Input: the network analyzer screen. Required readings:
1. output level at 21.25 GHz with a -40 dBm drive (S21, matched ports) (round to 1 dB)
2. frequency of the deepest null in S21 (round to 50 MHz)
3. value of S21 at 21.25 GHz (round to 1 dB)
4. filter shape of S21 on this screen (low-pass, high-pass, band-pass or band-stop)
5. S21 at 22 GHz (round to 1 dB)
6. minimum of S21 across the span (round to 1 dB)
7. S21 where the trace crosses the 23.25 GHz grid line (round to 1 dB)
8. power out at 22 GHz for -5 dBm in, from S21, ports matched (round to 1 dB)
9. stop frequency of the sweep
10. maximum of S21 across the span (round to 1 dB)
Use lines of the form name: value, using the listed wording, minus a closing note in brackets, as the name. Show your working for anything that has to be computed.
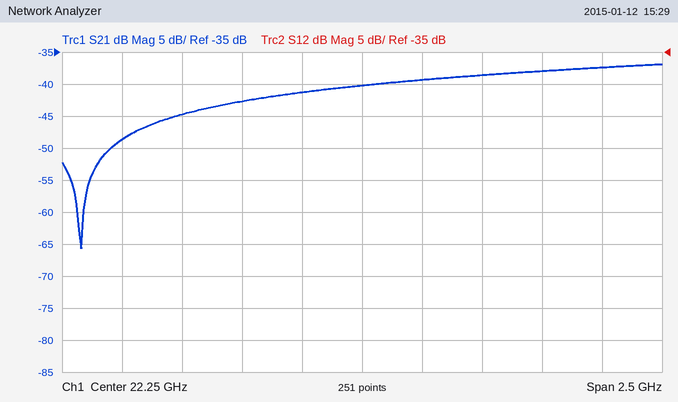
output level at 21.25 GHz with a -40 dBm drive (S21, matched ports): -40 dBm + (-49 dB) = -89 dBm
frequency of the deepest null in S21: 21.10 GHz
value of S21 at 21.25 GHz: -49 dB
filter shape of S21 on this screen: high-pass
S21 at 22 GHz: -41 dB
minimum of S21 across the span: -66 dB
S21 where the trace crosses the 23.25 GHz grid line: -37 dB
power out at 22 GHz for -5 dBm in, from S21, ports matched: -5 dBm + (-41 dB) = -46 dBm
stop frequency of the sweep: 23.5 GHz
maximum of S21 across the span: -37 dB
